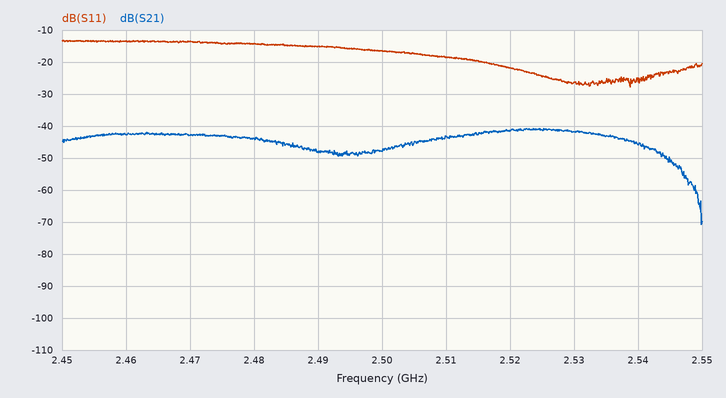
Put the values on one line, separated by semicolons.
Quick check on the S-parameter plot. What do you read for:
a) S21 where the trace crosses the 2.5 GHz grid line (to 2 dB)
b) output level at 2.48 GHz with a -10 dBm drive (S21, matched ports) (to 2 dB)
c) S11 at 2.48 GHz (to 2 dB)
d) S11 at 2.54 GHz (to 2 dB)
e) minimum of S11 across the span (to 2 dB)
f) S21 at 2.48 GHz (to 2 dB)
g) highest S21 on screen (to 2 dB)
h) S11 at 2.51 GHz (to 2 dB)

-48 dB; -54 dBm; -14 dB; -26 dB; -28 dB; -44 dB; -40 dB; -18 dB
